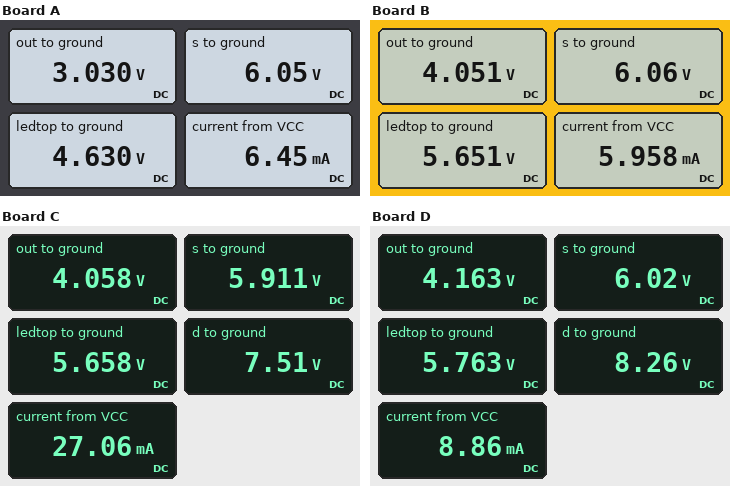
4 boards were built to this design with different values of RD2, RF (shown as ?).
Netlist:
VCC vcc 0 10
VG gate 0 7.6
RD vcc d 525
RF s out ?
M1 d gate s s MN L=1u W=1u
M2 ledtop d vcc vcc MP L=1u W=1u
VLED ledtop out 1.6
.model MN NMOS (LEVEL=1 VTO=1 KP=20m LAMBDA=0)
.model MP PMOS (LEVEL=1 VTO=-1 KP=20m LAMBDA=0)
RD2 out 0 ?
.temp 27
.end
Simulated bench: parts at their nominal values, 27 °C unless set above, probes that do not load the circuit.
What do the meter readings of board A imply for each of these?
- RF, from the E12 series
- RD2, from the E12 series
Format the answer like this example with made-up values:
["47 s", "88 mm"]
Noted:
["1 kΩ", "470 Ω"]
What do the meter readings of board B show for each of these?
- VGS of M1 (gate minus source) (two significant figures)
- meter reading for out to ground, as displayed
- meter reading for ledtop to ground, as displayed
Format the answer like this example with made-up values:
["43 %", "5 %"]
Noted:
["1.5 V", "4.051 V", "5.651 V"]
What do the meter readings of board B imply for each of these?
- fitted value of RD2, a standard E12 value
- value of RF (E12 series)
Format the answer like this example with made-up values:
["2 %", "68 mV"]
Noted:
["680 Ω", "680 Ω"]
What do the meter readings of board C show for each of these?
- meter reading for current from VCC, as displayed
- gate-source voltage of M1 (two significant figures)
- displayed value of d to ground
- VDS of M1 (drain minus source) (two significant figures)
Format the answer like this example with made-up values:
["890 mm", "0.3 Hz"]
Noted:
["27.06 mA", "1.7 V", "7.51 V", "1.6 V"]
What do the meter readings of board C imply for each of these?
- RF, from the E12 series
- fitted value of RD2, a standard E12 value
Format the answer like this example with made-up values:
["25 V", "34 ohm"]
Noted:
["390 Ω", "150 Ω"]
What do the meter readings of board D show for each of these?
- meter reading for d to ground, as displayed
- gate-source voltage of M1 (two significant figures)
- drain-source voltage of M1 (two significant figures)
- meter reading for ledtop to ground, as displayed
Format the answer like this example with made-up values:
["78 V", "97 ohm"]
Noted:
["8.26 V", "1.6 V", "2.2 V", "5.763 V"]
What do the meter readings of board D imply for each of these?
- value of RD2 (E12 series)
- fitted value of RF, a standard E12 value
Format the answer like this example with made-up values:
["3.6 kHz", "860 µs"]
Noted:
["470 Ω", "560 Ω"]
